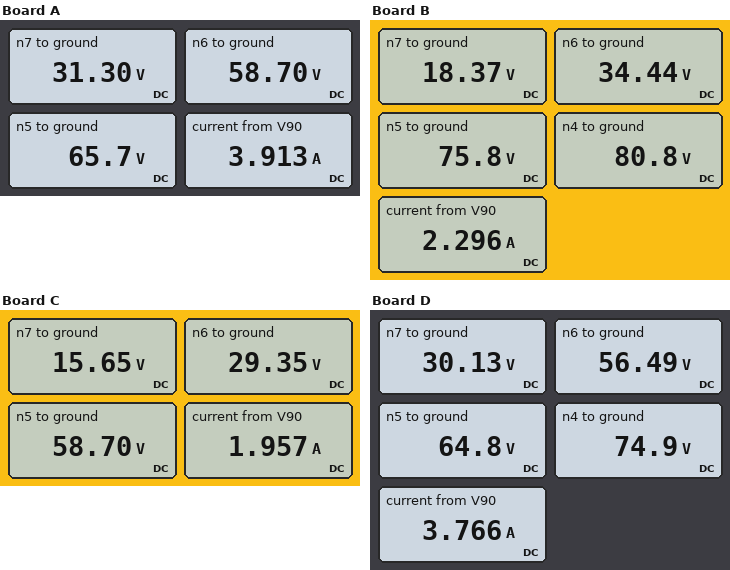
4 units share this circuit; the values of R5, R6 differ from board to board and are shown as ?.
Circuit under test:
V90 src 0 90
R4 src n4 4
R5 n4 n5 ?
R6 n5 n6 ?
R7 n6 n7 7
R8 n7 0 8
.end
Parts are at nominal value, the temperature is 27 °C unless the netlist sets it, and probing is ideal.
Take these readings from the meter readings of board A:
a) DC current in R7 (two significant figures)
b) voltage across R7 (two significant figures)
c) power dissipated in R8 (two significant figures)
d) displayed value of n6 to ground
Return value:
3.9 A
27 V
120 W
58.70 V
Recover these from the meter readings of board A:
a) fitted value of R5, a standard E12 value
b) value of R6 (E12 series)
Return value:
2.2 Ω
1.8 Ω
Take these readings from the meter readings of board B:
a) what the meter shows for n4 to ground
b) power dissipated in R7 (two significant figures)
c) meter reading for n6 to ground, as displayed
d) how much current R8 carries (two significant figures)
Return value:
80.8 V
37 W
34.44 V
2.3 A
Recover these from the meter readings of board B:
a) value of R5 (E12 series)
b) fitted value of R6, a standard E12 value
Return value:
2.2 Ω
18 Ω
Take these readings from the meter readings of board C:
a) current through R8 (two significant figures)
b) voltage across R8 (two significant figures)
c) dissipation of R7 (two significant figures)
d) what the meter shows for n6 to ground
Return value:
2.0 A
16 V
27 W
29.35 V
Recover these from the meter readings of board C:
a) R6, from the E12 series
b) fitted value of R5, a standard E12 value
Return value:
15 Ω
12 Ω
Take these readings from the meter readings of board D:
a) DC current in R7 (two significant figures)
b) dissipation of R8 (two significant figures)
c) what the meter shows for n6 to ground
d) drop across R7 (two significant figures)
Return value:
3.8 A
110 W
56.49 V
26 V
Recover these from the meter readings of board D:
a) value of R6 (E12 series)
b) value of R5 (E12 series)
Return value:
2.2 Ω
2.7 Ω
